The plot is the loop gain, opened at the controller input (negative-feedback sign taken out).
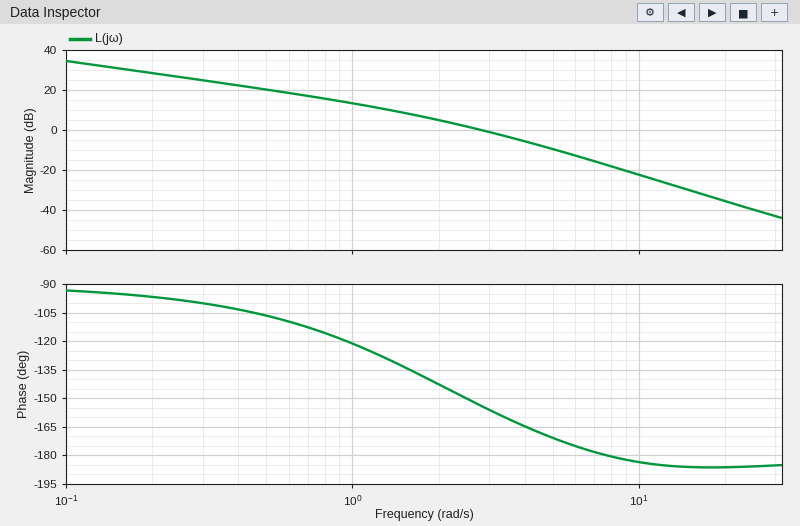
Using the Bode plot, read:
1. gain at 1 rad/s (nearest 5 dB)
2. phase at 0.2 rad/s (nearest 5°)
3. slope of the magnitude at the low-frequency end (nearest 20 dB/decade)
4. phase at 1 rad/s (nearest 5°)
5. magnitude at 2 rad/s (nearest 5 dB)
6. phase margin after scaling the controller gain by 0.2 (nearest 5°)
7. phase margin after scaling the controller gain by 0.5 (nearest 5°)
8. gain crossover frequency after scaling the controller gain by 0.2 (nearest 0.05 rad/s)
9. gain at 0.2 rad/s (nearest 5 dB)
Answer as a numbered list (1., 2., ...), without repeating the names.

1. 15 dB
2. -95°
3. -20 dB/decade
4. -120°
5. 5 dB
6. 60°
7. 40°
8. 0.95 rad/s
9. 30 dB
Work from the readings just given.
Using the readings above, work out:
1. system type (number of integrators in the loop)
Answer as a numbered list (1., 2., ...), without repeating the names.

1. 1
